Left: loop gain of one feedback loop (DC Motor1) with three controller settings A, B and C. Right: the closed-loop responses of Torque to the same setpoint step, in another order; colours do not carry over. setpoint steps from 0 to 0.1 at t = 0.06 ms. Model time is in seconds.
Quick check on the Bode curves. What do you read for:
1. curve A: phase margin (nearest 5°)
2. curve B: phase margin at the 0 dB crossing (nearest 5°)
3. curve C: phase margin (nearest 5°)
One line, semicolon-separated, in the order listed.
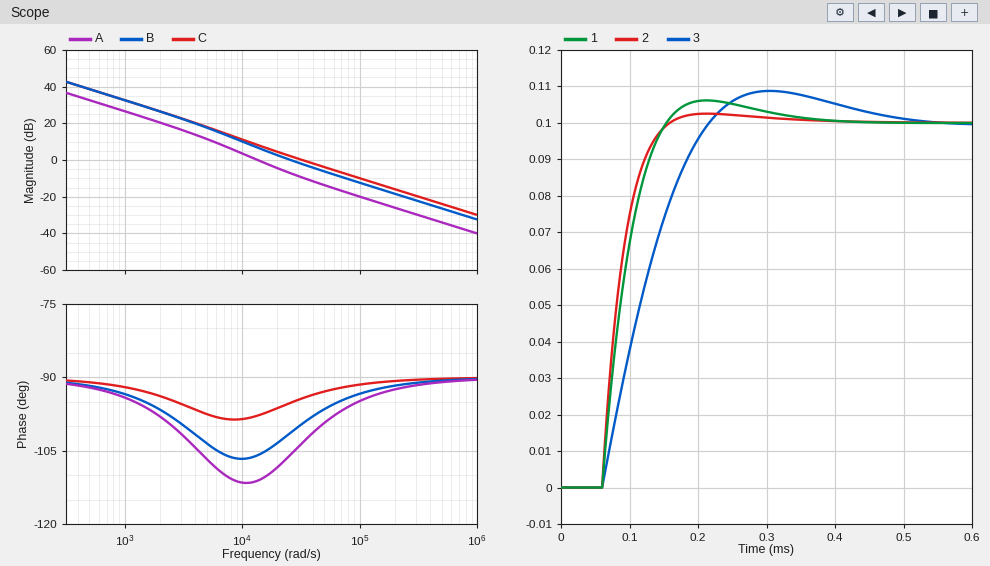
70°; 80°; 85°
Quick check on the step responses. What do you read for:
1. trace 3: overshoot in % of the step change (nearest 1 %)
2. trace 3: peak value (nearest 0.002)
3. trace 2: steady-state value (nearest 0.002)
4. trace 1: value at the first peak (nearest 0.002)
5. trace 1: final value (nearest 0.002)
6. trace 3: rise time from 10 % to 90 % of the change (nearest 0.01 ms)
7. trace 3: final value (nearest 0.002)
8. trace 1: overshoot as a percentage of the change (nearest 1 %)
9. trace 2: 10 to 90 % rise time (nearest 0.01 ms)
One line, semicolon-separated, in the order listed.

9 %; 0.108; 0.100; 0.106; 0.100; 0.11 ms; 0.100; 6 %; 0.06 ms
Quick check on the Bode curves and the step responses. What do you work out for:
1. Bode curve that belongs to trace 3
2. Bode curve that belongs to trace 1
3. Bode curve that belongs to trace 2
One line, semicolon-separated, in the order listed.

A; B; C
